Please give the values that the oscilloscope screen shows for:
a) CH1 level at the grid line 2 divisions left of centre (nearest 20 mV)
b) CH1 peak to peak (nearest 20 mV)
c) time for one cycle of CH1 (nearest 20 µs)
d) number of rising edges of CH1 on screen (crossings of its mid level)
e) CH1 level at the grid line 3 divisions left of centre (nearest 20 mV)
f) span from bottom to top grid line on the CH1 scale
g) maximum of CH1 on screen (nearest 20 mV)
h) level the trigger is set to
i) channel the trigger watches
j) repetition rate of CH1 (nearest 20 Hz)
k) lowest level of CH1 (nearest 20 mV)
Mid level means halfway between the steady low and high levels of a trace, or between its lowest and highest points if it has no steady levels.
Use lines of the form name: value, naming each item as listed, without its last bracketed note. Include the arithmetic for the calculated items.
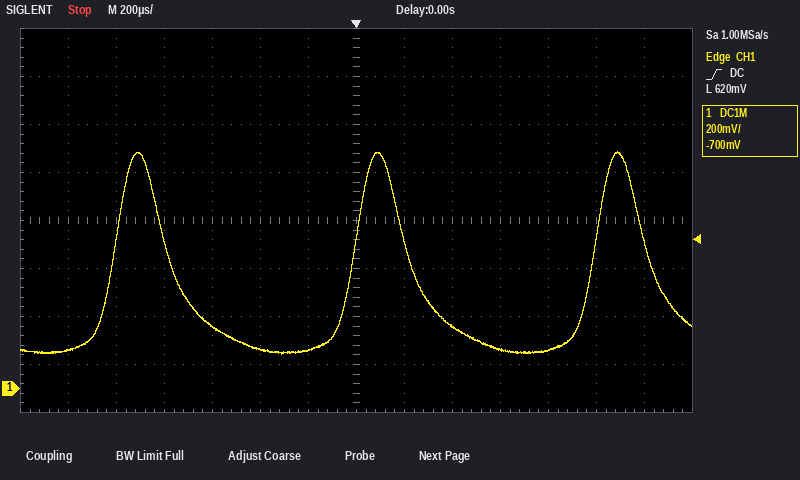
CH1 level at the grid line 2 divisions left of centre: 160 mV
CH1 peak to peak: 980 mV − (140 mV) = 840 mV
time for one cycle of CH1: 1.00 ms
number of rising edges of CH1 on screen: 3
CH1 level at the grid line 3 divisions left of centre: 260 mV
span from bottom to top grid line on the CH1 scale: 1.6 V
maximum of CH1 on screen: 980 mV
level the trigger is set to: 620 mV
channel the trigger watches: CH1
repetition rate of CH1: 1 / 1.00 ms ≈ 1.00 kHz
lowest level of CH1: 140 mV
